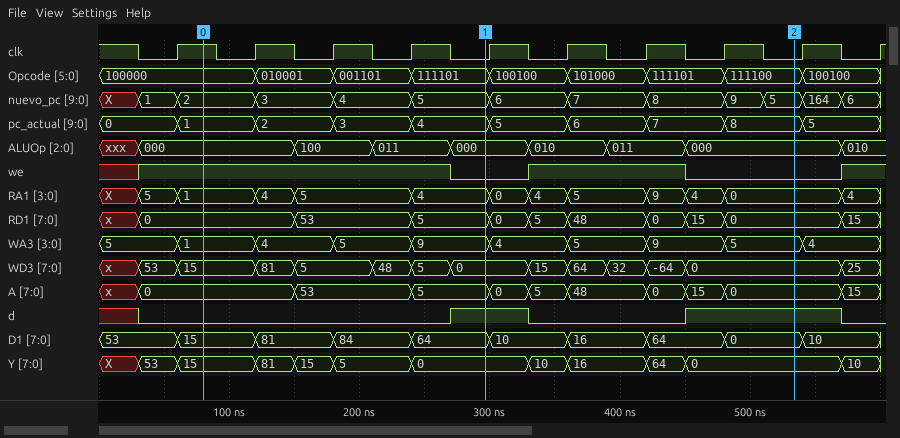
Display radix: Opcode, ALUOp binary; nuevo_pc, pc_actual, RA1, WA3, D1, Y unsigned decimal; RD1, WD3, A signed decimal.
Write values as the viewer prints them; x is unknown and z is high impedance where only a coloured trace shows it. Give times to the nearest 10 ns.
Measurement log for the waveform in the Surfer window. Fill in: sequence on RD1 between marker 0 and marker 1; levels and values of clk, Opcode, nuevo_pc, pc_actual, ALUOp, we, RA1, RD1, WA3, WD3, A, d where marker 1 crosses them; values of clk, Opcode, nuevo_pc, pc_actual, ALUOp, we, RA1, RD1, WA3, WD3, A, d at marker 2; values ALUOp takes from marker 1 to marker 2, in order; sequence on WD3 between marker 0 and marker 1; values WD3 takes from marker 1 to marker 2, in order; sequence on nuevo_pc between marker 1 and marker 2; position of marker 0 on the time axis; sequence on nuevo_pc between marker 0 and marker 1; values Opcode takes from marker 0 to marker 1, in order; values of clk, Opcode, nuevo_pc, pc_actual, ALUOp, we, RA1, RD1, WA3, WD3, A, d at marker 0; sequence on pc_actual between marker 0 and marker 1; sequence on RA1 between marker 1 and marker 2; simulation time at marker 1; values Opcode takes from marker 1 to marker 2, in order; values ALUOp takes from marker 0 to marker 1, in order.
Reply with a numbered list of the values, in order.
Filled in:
1. 0, 53, 5
2. clk=0, Opcode=111101, nuevo_pc=5, pc_actual=4, ALUOp=000, we=0, RA1=4, RD1=5, WA3=9, WD3=0, A=5, d=1
3. clk=0, Opcode=111100, nuevo_pc=5, pc_actual=8, ALUOp=000, we=0, RA1=0, RD1=0, WA3=5, WD3=0, A=0, d=1
4. 000, 010, 011, 000
5. 15, 81, 5, 48, 5, 0
6. 0, 15, 64, 32, -64, 0
7. 5, 6, 7, 8, 9, 5
8. 80 ns
9. 2, 3, 4, 5
10. 100000, 010001, 001101, 111101
11. clk=1, Opcode=100000, nuevo_pc=2, pc_actual=1, ALUOp=000, we=1, RA1=1, RD1=0, WA3=1, WD3=15, A=0, d=0
12. 1, 2, 3, 4
13. 4, 0, 4, 5, 9, 4, 0
14. 300 ns
15. 111101, 100100, 101000, 111101, 111100
16. 000, 100, 011, 000
